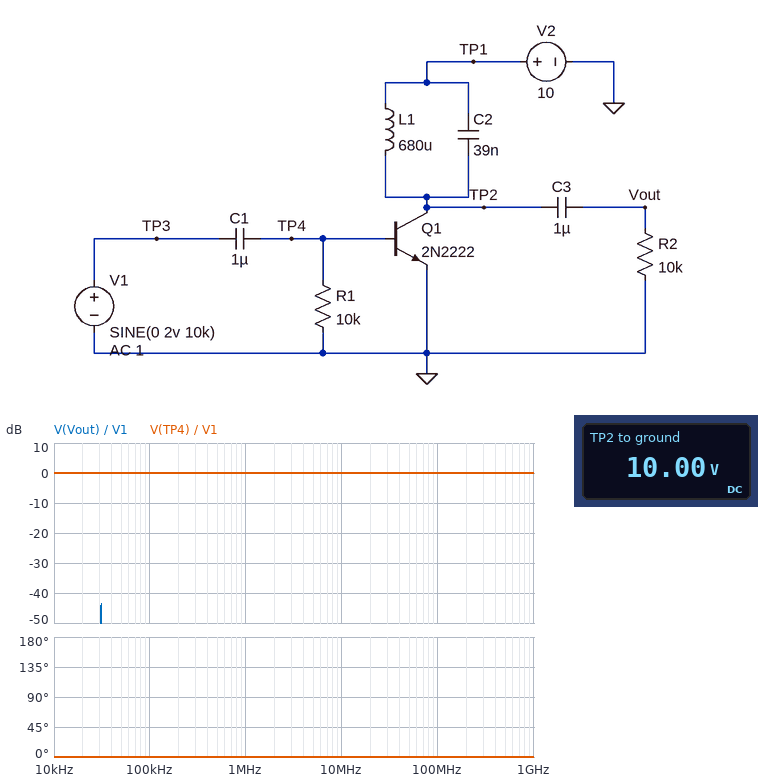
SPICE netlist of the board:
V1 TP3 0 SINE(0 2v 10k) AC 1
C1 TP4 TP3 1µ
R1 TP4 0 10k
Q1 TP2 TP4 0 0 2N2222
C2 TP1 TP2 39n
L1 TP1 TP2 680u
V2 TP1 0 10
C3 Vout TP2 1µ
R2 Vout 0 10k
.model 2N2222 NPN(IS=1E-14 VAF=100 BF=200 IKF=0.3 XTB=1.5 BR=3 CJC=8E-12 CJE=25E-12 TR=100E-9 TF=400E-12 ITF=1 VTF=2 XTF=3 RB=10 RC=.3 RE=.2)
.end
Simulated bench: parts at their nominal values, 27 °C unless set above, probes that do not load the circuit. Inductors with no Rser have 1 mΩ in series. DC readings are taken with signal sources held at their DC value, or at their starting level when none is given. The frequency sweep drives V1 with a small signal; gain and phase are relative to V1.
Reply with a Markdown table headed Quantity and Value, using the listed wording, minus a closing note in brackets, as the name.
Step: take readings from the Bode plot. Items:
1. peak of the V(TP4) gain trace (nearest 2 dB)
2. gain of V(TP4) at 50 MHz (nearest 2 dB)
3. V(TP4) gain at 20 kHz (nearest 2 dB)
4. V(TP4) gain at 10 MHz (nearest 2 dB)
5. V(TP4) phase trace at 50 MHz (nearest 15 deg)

| Quantity | Value |
|---|---|
| peak of the V(TP4) gain trace | 0 dB |
| gain of V(TP4) at 50 MHz | 0 dB |
| V(TP4) gain at 20 kHz | 0 dB |
| V(TP4) gain at 10 MHz | 0 dB |
| V(TP4) phase trace at 50 MHz | 0 deg |
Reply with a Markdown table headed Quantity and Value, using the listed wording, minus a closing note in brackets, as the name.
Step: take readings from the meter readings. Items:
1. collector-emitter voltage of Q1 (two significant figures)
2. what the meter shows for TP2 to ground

| Quantity | Value |
|---|---|
| collector-emitter voltage of Q1 | 10 V |
| what the meter shows for TP2 to ground | 10.00 V |
